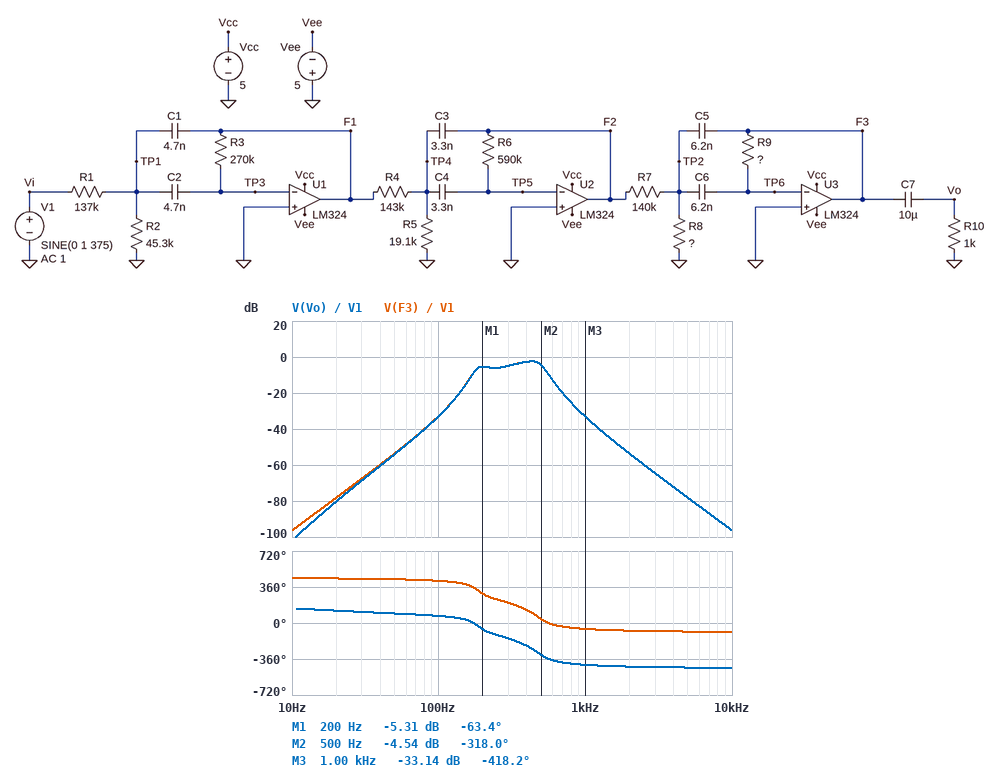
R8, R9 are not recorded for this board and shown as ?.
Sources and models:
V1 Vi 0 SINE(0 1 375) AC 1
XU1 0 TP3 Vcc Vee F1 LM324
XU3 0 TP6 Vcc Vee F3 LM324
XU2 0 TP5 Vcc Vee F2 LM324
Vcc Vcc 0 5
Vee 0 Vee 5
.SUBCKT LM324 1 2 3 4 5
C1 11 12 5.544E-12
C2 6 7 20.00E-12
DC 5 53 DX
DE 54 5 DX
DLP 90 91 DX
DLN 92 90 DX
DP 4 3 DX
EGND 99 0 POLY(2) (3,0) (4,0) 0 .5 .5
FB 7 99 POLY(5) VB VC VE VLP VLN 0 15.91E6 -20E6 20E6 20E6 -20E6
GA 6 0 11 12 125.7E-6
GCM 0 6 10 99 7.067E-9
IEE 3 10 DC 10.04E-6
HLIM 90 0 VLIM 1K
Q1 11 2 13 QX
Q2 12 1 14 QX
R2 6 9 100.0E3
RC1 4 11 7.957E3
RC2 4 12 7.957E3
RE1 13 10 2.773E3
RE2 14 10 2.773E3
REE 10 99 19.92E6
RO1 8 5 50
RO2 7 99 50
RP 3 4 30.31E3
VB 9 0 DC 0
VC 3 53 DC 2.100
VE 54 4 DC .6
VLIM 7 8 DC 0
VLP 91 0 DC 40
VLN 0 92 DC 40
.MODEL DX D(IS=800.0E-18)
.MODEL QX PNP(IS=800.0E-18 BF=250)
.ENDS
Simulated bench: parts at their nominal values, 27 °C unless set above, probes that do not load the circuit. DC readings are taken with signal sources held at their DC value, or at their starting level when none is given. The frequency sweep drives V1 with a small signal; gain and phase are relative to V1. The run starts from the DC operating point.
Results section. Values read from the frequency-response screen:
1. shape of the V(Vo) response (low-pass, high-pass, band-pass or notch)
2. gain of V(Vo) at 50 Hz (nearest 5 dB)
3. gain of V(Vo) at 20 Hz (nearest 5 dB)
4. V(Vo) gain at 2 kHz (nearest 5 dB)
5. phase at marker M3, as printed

band-pass
-55 dB
-80 dB
-55 dB
-418.2 deg
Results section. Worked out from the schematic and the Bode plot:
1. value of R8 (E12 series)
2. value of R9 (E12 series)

22 kΩ
1 MΩ
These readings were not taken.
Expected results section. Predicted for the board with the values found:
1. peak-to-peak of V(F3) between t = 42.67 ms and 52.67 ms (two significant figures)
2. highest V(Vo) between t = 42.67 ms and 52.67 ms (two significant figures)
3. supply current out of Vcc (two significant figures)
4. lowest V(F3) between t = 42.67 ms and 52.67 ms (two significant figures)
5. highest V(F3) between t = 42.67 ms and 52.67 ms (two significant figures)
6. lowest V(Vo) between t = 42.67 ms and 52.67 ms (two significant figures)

1.4 V
700 mV
1.0 mA
-720 mV
680 mV
-700 mV
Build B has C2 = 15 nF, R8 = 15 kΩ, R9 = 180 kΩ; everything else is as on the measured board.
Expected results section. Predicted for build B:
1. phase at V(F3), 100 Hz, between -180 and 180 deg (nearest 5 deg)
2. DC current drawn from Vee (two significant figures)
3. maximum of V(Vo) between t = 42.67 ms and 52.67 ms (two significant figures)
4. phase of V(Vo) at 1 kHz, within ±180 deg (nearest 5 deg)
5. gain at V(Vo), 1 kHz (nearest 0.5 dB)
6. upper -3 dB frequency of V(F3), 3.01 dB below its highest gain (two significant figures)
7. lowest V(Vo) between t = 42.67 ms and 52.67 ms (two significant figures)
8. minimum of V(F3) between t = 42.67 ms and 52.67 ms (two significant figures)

50 deg
1.0 mA
360 mV
-45 deg
-32.0 dB
550 Hz
-360 mV
-370 mV
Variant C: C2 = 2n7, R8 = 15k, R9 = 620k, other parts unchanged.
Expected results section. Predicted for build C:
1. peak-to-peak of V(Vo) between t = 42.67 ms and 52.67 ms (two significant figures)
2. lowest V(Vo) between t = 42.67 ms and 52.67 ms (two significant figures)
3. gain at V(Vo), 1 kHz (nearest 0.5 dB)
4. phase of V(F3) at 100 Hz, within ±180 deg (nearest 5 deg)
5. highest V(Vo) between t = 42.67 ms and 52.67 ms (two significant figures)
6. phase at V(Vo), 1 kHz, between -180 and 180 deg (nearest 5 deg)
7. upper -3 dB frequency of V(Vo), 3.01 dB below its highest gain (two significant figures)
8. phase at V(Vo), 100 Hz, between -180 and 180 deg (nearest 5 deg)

1.4 V
-690 mV
-32.0 dB
70 deg
690 mV
-50 deg
520 Hz
80 deg
